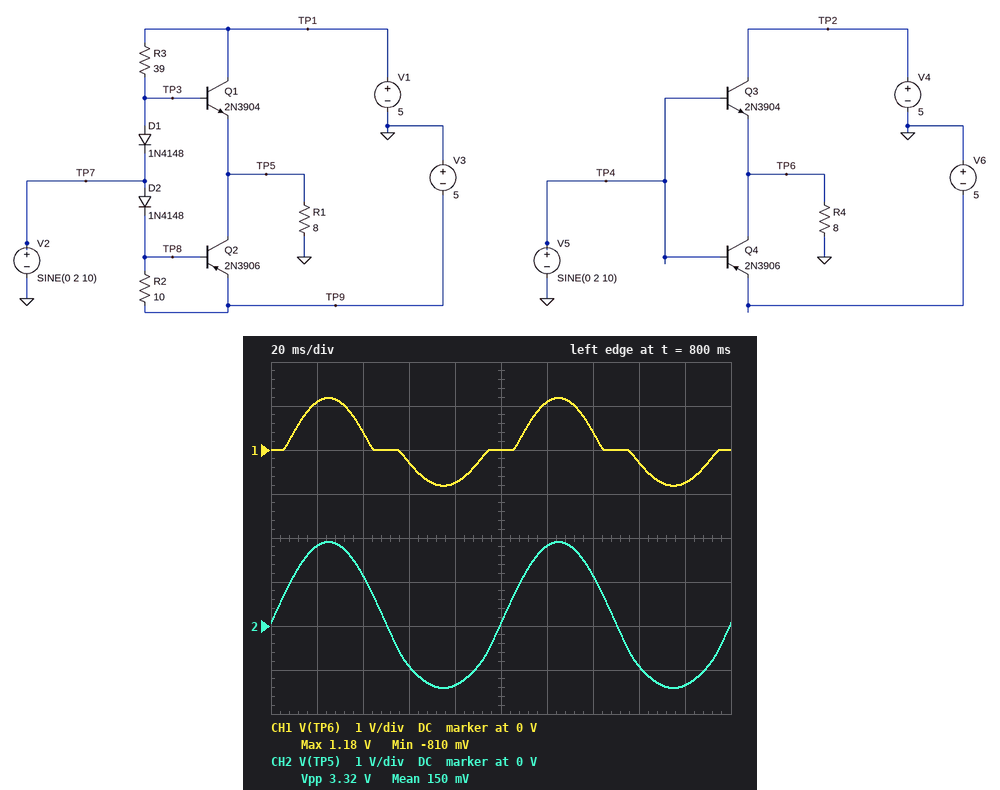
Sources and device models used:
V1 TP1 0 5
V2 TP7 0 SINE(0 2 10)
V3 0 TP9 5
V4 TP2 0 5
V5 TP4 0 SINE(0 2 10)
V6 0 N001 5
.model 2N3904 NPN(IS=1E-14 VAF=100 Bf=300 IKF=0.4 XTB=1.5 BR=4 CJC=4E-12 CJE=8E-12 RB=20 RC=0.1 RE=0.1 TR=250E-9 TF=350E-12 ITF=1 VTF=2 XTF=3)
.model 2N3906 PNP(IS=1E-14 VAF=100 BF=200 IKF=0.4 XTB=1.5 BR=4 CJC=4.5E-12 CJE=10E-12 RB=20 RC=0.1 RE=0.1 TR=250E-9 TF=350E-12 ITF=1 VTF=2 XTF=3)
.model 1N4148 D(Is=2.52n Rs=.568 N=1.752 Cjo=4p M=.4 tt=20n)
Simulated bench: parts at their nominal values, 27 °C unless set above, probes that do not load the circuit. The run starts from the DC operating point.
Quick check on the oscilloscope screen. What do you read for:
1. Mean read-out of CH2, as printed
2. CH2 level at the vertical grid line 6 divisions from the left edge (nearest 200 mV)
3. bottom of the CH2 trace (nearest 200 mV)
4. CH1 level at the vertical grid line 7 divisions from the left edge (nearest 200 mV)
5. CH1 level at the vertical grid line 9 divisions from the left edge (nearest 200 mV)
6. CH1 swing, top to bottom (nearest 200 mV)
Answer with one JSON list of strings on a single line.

["150 mV", "1.8 V", "-1.4 V", "400 mV", "-800 mV", "2.0 V"]
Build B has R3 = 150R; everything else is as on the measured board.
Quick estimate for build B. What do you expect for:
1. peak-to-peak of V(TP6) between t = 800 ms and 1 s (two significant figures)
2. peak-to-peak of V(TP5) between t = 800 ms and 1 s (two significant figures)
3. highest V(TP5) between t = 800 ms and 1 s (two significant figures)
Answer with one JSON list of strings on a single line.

["2.0 V", "3.2 V", "1.8 V"]
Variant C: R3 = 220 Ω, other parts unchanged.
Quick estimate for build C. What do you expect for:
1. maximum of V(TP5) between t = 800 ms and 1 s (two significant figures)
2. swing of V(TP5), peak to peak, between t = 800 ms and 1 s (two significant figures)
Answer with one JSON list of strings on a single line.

["1.8 V", "3.2 V"]
